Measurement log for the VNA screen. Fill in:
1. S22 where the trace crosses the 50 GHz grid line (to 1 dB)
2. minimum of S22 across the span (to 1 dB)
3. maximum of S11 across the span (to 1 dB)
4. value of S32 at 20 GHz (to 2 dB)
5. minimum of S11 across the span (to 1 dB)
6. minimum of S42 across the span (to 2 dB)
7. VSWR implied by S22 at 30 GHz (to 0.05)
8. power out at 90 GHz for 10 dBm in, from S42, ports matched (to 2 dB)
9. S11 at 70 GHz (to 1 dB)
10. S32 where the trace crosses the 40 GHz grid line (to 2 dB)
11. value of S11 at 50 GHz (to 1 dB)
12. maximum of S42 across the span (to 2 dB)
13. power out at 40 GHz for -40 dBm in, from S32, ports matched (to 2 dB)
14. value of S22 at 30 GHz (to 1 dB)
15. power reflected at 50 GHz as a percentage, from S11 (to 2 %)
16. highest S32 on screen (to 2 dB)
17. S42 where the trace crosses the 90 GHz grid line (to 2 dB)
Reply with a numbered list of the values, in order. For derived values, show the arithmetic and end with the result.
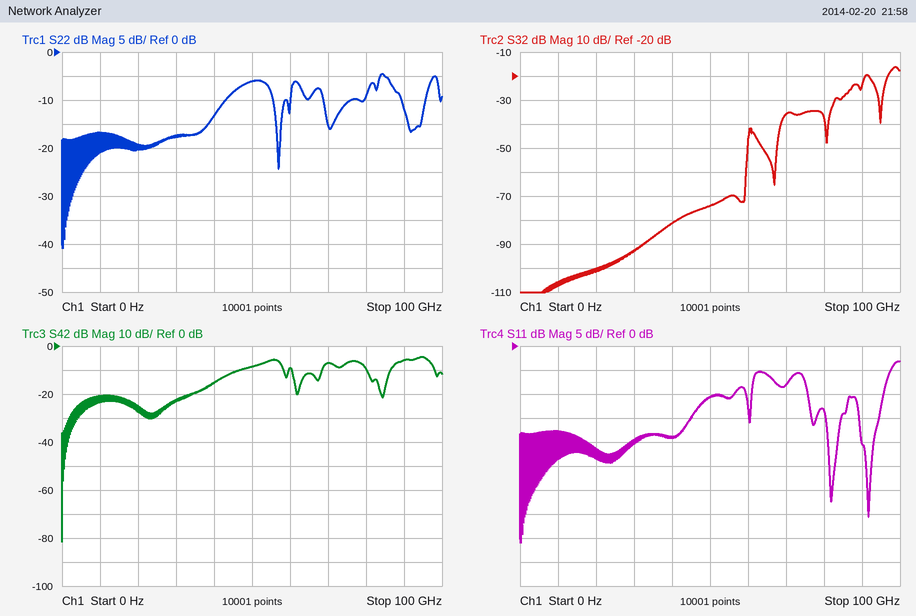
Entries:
1. -6 dB
2. -41 dB
3. -3 dB
4. -100 dB
5. -41 dB
6. -82 dB
7. |Γ| = 10^(-18/20) = 0.1259; VSWR = (1 + 0.1259)/(1 − 0.1259) ≈ 1.29, so 1.30 to the nearest 0.05
8. 10 dBm + (-6 dB) = 4 dBm
9. -8 dB
10. -82 dB
11. -11 dB
12. -4 dB
13. -40 dBm + (-82 dB) = -122 dBm
14. -18 dB
15. 10^(-11/10) ≈ 8 %
16. -16 dB
17. -6 dB
